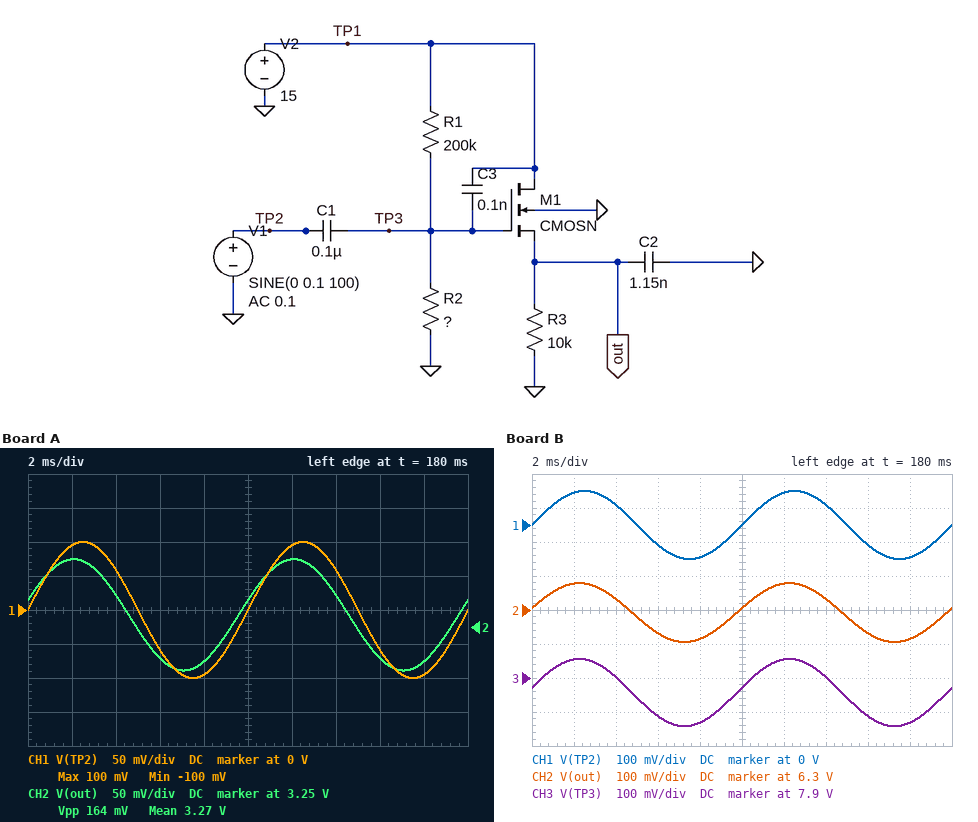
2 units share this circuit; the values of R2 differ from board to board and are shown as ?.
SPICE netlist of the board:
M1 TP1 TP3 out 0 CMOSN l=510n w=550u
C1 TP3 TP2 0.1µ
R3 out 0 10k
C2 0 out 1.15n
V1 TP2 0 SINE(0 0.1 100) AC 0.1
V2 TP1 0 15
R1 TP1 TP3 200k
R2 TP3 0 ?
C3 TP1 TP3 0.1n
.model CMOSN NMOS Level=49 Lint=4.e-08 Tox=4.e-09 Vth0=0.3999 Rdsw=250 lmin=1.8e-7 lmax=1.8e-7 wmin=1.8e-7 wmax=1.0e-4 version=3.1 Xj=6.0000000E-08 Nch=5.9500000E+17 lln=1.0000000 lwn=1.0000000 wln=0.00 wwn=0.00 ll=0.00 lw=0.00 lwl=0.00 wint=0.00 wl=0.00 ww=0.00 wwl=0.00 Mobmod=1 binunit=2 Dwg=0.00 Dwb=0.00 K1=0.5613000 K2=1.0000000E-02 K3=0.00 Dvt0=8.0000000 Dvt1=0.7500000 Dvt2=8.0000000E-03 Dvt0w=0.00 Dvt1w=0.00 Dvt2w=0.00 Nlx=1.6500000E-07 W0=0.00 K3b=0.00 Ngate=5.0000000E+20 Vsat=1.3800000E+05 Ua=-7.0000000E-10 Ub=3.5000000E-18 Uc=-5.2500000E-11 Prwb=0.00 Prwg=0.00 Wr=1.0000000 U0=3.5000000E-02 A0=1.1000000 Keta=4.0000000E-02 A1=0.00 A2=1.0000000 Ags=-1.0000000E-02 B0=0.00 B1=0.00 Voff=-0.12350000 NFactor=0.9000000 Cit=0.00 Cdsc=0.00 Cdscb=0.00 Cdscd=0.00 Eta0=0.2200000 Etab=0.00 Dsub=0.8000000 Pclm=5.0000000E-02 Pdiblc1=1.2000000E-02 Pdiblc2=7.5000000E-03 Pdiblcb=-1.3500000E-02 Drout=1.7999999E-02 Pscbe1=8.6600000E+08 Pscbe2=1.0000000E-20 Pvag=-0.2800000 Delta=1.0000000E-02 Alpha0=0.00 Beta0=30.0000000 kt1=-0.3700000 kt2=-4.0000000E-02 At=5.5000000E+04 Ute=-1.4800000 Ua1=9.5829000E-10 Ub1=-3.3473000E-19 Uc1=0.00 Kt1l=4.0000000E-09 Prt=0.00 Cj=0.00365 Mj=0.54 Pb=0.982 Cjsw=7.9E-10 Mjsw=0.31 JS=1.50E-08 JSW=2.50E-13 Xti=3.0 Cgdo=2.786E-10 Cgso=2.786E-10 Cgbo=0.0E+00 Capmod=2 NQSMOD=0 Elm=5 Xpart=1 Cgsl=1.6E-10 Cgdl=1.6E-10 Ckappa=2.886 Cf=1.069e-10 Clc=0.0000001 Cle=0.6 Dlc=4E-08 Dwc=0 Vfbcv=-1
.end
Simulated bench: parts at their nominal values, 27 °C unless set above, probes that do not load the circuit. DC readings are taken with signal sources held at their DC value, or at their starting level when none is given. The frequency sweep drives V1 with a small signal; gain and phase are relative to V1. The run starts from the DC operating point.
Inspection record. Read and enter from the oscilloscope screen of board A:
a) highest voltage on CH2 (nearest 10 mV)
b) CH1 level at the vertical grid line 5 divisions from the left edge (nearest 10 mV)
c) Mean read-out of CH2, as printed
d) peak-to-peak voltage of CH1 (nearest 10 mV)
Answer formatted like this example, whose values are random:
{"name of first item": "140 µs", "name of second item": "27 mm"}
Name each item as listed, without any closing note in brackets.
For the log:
{"highest voltage on CH2": "3.35 V", "CH1 level at the vertical grid line 5 divisions from the left edge": "0 V", "Mean read-out of CH2, as printed": "3.27 V", "peak-to-peak voltage of CH1": "200 mV"}
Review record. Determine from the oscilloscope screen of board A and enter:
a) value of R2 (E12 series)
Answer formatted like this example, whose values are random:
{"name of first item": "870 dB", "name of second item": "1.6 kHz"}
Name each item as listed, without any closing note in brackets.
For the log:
{"value of R2": "82 kΩ"}
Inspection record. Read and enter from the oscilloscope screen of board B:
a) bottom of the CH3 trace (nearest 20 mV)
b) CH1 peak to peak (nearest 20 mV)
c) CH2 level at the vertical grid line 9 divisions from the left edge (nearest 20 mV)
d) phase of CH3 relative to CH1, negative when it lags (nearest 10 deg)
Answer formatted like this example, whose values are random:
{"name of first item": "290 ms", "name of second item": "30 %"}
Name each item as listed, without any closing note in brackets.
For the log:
{"bottom of the CH3 trace": "7.76 V", "CH1 peak to peak": "200 mV", "CH2 level at the vertical grid line 9 divisions from the left edge": "6.22 V", "phase of CH3 relative to CH1, negative when it lags": "10 deg"}
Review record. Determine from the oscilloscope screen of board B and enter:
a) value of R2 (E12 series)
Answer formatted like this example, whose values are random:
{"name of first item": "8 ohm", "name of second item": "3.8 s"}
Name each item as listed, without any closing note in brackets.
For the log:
{"value of R2": "220 kΩ"}
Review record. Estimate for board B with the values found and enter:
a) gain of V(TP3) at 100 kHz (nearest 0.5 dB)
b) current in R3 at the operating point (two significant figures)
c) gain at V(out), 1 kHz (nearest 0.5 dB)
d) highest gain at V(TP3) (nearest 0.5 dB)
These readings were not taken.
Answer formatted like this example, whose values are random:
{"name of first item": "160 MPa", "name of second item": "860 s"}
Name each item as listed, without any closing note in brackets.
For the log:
{"gain of V(TP3) at 100 kHz": "0 dB", "current in R3 at the operating point": "630 µA", "gain at V(out), 1 kHz": "-1.0 dB", "highest gain at V(TP3)": "0 dB"}
